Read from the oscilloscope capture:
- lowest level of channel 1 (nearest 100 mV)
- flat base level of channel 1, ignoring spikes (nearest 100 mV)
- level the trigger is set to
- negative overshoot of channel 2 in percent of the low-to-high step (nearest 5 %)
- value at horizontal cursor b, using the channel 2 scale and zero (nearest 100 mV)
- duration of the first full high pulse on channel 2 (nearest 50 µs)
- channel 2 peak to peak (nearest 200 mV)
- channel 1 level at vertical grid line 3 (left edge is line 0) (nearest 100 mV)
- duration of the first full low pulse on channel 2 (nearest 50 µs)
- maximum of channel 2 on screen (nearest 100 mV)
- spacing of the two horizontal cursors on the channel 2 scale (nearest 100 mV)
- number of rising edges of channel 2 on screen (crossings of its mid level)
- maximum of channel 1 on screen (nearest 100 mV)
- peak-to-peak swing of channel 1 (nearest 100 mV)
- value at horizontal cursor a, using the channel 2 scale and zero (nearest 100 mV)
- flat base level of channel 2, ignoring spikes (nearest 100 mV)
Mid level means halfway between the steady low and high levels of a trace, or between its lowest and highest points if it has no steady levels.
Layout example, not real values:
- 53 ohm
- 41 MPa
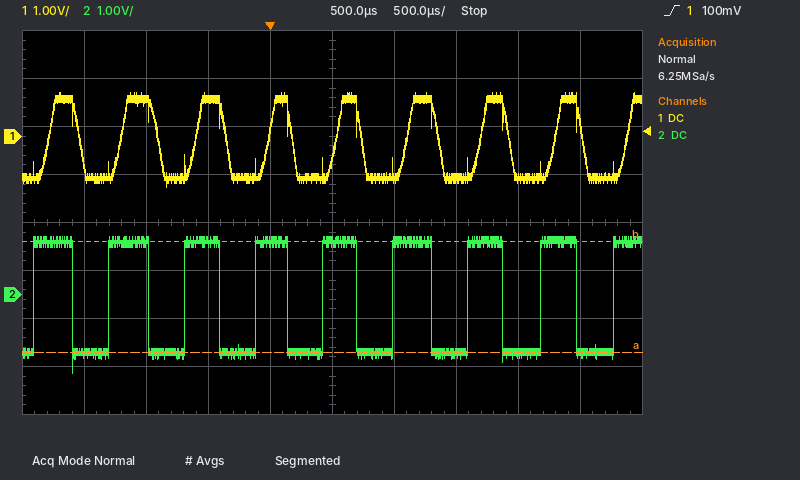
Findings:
- -1.1 V
- -900 mV
- 100 mV
- 20 %
- 1.1 V
- 300 µs
- 2.8 V
- 800 mV
- 300 µs
- 1.2 V
- 2.3 V
- 9
- 900 mV
- 2.0 V
- -1.2 V
- -1.2 V
